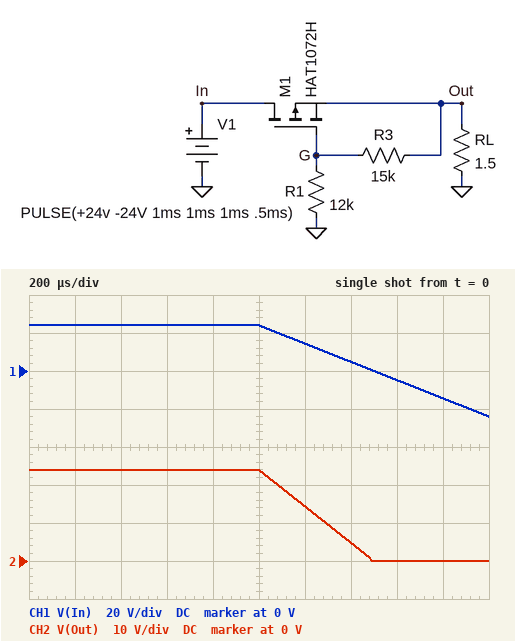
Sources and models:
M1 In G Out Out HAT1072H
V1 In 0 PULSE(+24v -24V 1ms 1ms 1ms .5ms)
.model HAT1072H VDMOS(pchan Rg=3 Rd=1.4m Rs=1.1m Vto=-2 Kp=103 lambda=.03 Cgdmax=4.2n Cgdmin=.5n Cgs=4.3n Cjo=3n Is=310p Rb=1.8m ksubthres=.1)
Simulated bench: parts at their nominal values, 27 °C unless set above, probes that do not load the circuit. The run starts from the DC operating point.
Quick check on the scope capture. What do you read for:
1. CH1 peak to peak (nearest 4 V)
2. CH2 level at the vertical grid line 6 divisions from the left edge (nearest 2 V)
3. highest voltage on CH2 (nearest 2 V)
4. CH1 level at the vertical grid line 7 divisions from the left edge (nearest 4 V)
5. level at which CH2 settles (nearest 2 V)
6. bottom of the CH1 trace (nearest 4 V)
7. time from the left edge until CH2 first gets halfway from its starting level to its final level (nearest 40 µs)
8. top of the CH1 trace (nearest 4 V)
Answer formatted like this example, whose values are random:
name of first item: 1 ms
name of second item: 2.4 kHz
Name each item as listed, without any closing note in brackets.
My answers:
CH1 peak to peak: 48 V
CH2 level at the vertical grid line 6 divisions from the left edge: 14 V
highest voltage on CH2: 24 V
CH1 level at the vertical grid line 7 divisions from the left edge: 4 V
level at which CH2 settles: 0 V
bottom of the CH1 trace: -24 V
time from the left edge until CH2 first gets halfway from its starting level to its final level: 1.24 ms
top of the CH1 trace: 24 V
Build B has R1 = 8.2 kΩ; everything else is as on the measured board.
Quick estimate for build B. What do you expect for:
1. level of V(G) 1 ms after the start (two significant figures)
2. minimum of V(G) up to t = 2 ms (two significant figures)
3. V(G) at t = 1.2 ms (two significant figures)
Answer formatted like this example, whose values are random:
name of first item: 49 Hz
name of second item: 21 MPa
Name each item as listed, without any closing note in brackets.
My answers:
level of V(G) 1 ms after the start: 8.5 V
minimum of V(G) up to t = 2 ms: -1.4 V
V(G) at t = 1.2 ms: 3.7 V
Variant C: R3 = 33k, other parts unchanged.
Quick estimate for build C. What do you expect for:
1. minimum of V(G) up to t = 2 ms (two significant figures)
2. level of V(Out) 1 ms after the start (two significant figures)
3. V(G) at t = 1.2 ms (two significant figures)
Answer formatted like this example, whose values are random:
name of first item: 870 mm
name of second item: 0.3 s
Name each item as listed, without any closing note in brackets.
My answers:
minimum of V(G) up to t = 2 ms: -2.8 V
level of V(Out) 1 ms after the start: 24 V
V(G) at t = 1.2 ms: 1.4 V
